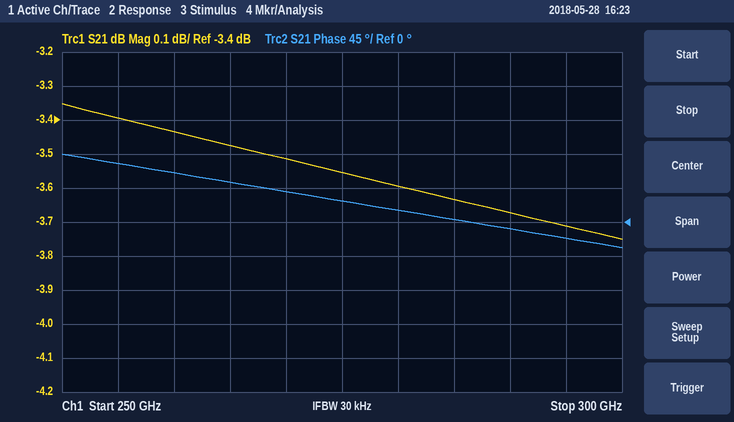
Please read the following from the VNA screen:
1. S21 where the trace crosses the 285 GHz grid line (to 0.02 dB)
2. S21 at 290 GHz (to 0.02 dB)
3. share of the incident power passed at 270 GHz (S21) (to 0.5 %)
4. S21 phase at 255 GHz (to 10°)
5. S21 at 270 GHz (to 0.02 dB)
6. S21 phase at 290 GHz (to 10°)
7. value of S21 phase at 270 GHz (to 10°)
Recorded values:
-3.64 dB
-3.68 dB
44.5 %
80°
-3.52 dB
-10°
40°
